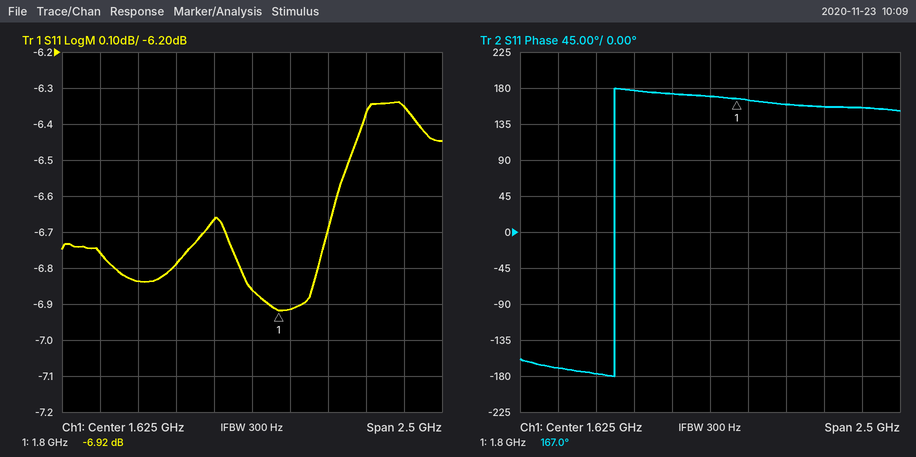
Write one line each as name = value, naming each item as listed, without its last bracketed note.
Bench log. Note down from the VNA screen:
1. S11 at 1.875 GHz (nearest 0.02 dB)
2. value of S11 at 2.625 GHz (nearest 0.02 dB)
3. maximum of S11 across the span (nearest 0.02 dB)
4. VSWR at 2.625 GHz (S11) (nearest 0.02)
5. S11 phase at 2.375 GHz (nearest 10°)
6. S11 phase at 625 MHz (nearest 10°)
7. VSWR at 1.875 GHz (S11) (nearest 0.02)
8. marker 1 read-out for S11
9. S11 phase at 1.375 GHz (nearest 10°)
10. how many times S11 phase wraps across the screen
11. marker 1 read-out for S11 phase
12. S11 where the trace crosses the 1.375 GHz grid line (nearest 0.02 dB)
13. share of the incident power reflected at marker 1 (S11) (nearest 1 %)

S11 at 1.875 GHz = -6.92 dB
value of S11 at 2.625 GHz = -6.36 dB
maximum of S11 across the span = -6.34 dB
VSWR at 2.625 GHz (S11) = 2.86
S11 phase at 2.375 GHz = 160°
S11 phase at 625 MHz = -170°
VSWR at 1.875 GHz (S11) = 2.64
marker 1 read-out for S11 = -6.92 dB
S11 phase at 1.375 GHz = 170°
how many times S11 phase wraps across the screen = 1
marker 1 read-out for S11 phase = 167.0°
S11 where the trace crosses the 1.375 GHz grid line = -6.66 dB
share of the incident power reflected at marker 1 (S11) = 20 %
